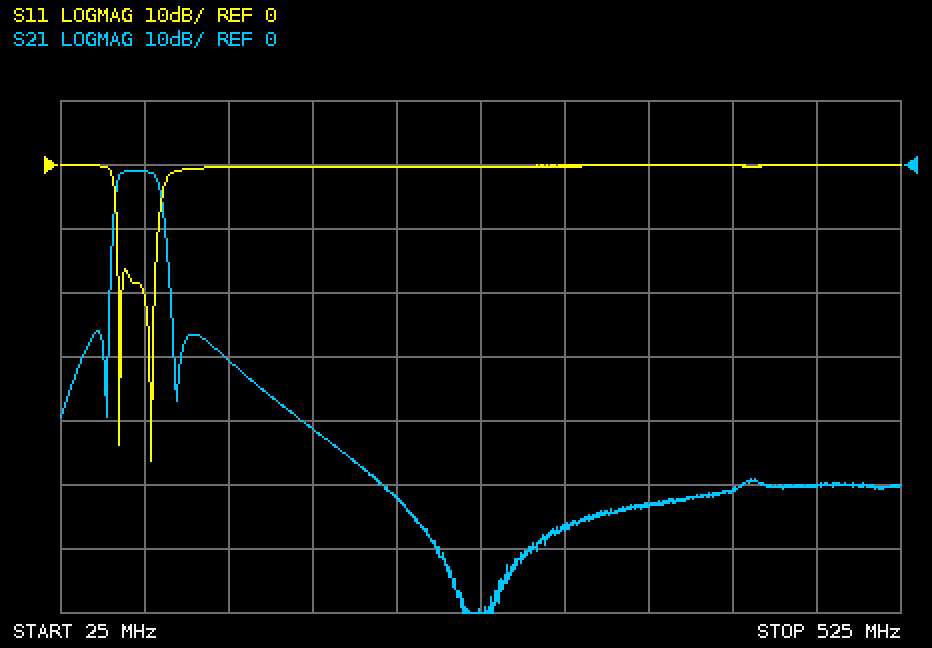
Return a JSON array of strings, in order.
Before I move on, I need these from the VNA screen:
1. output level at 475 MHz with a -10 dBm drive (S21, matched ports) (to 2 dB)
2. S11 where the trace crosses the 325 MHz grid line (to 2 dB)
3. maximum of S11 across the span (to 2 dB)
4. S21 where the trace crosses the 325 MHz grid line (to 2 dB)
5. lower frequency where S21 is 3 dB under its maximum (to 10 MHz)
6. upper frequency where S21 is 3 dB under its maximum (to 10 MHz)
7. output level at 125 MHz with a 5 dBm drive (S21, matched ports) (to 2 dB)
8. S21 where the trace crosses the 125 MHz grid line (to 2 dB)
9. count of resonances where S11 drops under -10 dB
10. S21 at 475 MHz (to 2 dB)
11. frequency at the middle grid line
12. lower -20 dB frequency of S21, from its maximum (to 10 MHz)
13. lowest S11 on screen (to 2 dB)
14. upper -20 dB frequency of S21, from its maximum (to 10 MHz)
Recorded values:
["-60 dBm", "0 dB", "0 dB", "-56 dB", "60 MHz", "80 MHz", "-26 dBm", "-30 dB", "2", "-50 dB", "275 MHz", "50 MHz", "-46 dB", "90 MHz"]
